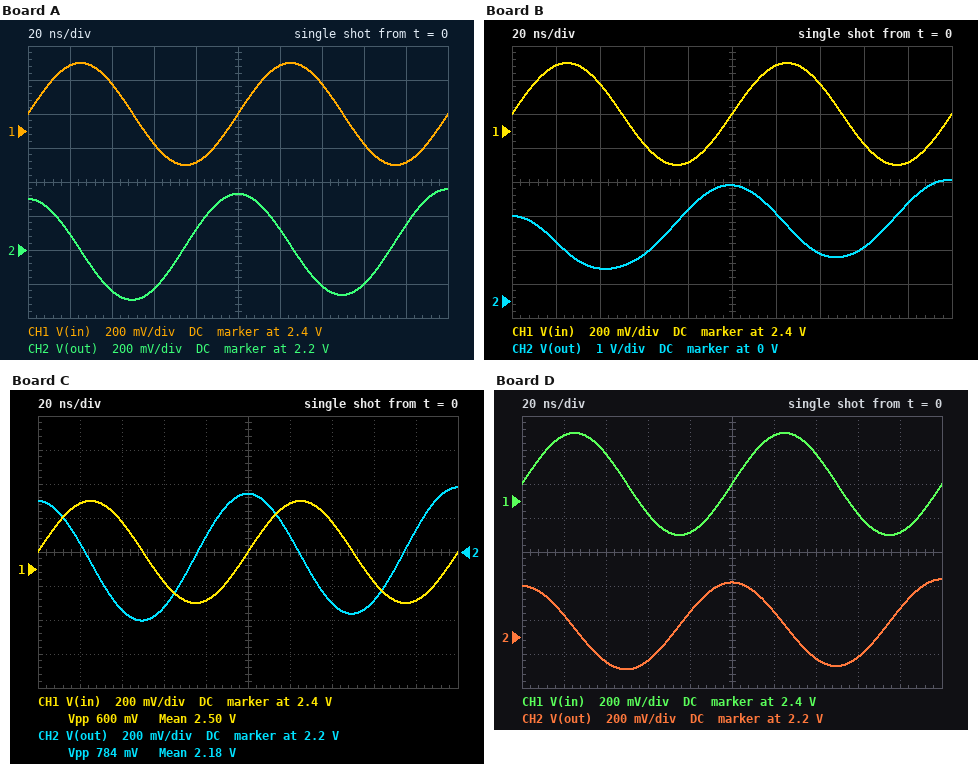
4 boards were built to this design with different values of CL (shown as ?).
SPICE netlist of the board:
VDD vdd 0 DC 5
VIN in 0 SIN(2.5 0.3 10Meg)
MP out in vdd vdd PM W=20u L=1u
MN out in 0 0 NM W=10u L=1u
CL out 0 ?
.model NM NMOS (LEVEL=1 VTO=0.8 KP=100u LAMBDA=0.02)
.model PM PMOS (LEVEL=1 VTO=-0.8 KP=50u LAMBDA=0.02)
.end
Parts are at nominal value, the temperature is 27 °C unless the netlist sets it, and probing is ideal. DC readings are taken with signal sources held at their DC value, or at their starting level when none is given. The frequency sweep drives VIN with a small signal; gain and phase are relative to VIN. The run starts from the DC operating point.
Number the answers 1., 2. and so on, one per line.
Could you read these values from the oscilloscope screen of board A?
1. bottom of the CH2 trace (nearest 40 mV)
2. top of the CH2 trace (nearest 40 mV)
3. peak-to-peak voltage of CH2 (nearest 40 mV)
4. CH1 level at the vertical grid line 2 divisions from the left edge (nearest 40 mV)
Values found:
1. 1.92 V
2. 2.56 V
3. 640 mV
4. 2.68 V
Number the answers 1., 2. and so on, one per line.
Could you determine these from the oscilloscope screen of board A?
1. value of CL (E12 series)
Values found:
1. 56 pF
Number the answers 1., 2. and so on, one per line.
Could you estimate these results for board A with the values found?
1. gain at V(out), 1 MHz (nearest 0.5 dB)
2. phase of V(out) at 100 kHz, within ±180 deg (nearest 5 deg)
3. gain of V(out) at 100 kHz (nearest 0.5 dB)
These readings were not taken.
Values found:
1. 20.0 dB
2. 150 deg
3. 34.5 dB
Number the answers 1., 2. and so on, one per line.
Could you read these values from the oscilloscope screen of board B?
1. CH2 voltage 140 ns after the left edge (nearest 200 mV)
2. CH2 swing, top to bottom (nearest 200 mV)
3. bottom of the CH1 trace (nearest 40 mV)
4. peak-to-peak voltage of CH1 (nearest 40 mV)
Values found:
1. 1.4 V
2. 2.6 V
3. 2.20 V
4. 600 mV
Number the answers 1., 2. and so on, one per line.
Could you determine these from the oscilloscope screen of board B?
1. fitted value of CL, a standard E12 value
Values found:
1. 15 pF
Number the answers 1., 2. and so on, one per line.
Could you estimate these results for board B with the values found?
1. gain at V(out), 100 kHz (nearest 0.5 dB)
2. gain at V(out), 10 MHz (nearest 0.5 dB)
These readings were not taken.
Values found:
1. 35.5 dB
2. 11.5 dB
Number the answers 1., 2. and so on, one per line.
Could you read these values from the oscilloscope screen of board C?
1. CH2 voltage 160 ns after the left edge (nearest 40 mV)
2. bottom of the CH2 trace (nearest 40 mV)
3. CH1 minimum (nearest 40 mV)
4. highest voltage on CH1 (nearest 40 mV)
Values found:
1. 1.92 V
2. 1.80 V
3. 2.20 V
4. 2.80 V
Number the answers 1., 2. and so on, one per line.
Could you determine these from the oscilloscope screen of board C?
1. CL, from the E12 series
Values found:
1. 47 pF
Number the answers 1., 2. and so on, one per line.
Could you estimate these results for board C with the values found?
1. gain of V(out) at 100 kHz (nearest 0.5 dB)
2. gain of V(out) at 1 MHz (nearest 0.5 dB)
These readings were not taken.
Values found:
1. 35.0 dB
2. 21.5 dB
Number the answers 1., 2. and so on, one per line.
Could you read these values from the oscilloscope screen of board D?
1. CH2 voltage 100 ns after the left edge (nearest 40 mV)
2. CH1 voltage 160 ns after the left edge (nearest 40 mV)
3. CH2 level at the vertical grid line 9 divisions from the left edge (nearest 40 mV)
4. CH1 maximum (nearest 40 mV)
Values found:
1. 2.52 V
2. 2.32 V
3. 2.36 V
4. 2.80 V
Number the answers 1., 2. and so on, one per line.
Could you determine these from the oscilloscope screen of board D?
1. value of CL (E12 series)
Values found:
1. 68 pF
